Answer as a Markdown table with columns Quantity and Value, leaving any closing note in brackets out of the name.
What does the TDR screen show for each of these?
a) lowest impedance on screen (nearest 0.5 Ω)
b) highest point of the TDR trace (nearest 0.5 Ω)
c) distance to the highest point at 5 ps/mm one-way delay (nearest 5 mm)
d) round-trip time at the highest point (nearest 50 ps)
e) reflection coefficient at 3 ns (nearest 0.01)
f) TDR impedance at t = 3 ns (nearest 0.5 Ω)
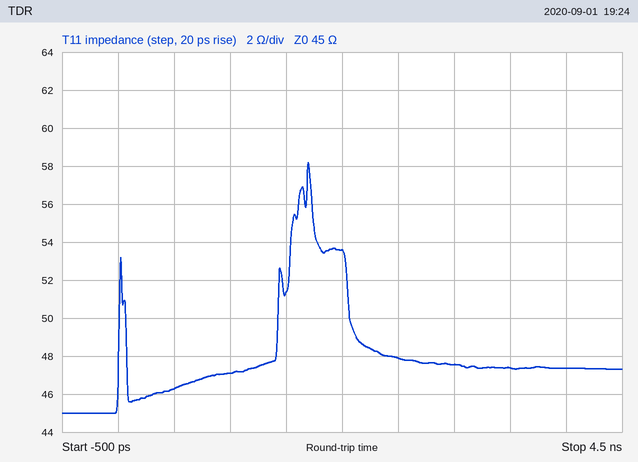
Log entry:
| Quantity | Value |
|---|---|
| lowest impedance on screen | 45.0 Ω |
| highest point of the TDR trace | 58.0 Ω |
| distance to the highest point at 5 ps/mm one-way delay | 170 mm |
| round-trip time at the highest point | 1.70 ns |
| reflection coefficient at 3 ns | +0.03 |
| TDR impedance at t = 3 ns | 47.5 Ω |
